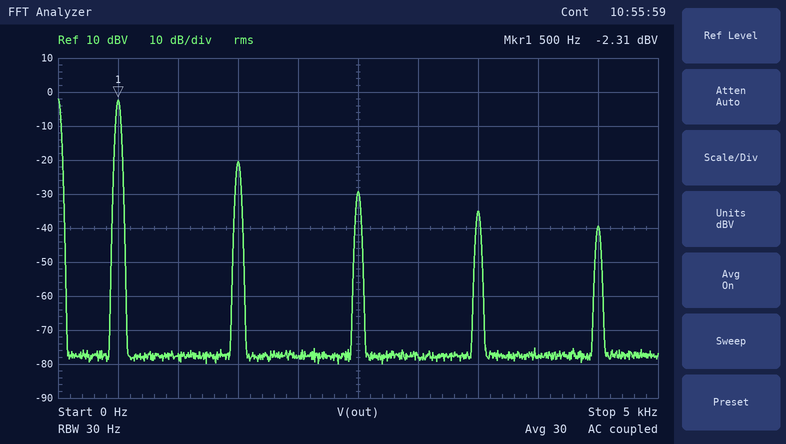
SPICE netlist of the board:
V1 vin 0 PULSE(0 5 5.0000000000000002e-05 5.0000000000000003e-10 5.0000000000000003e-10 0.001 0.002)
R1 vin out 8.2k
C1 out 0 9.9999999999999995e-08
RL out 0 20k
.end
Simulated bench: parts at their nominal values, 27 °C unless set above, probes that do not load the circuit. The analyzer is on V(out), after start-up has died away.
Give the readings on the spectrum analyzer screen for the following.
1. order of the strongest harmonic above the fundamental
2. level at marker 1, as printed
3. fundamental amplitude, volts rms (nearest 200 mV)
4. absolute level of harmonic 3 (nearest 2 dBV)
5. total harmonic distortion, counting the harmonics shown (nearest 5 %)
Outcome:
3
-2.31 dBV
800 mV
-20 dBV
15 %
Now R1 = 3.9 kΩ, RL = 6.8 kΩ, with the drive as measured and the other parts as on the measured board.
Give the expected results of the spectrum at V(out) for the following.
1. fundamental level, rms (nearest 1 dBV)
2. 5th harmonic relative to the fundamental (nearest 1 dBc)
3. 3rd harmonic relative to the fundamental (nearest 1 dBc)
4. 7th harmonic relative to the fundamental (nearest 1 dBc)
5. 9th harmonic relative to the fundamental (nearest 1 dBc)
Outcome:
1 dBV
-24 dBc
-16 dBc
-30 dBc
-34 dBc
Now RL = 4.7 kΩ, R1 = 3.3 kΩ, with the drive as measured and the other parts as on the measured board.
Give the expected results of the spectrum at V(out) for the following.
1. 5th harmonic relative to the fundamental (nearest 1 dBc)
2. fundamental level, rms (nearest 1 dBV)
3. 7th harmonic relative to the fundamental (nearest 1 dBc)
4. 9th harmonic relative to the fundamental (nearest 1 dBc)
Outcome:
-23 dBc
1 dBV
-28 dBc
-33 dBc
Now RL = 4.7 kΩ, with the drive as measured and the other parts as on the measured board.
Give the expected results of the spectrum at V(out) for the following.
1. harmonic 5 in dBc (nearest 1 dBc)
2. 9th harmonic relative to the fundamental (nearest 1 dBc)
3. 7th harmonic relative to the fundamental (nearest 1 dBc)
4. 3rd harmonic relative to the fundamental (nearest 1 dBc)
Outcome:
-25 dBc
-35 dBc
-31 dBc
-16 dBc
